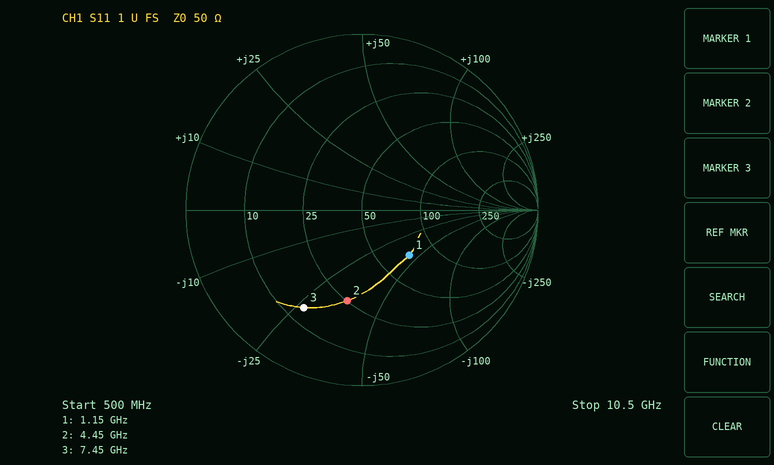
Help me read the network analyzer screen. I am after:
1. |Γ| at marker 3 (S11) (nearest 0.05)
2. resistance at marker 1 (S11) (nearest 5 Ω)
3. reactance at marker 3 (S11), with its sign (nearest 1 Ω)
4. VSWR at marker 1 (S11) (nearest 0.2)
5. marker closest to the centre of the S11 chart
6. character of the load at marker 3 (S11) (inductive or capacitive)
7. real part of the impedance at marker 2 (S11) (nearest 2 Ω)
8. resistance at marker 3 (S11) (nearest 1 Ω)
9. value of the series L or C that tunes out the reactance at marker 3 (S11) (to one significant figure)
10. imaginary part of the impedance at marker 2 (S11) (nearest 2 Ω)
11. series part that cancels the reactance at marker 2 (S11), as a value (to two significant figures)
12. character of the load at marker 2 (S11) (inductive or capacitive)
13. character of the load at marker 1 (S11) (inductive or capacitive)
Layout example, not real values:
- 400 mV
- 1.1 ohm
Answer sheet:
- 0.65
- 70 Ω
- -27 Ω
- 2.2
- marker 1
- capacitive
- 26 Ω
- 14 Ω
- 600 pH
- -36 Ω
- 1.3 nH
- capacitive
- capacitive
